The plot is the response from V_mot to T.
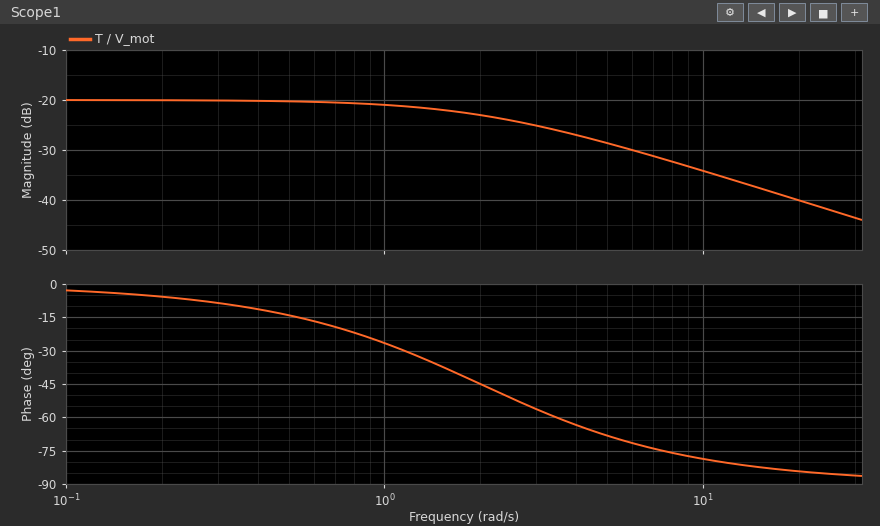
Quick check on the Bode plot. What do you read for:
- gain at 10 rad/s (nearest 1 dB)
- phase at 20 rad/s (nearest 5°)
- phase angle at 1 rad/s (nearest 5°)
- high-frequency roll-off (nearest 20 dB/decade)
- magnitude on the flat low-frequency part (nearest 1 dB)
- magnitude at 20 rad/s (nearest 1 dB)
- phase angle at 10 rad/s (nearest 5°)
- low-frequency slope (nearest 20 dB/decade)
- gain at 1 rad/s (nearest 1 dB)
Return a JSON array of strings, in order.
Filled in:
["-34 dB", "-85°", "-25°", "-20 dB/decade", "-20 dB", "-40 dB", "-80°", "0 dB/decade", "-21 dB"]
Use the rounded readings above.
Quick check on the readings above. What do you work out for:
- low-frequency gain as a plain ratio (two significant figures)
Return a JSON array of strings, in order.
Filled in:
["0.10"]
